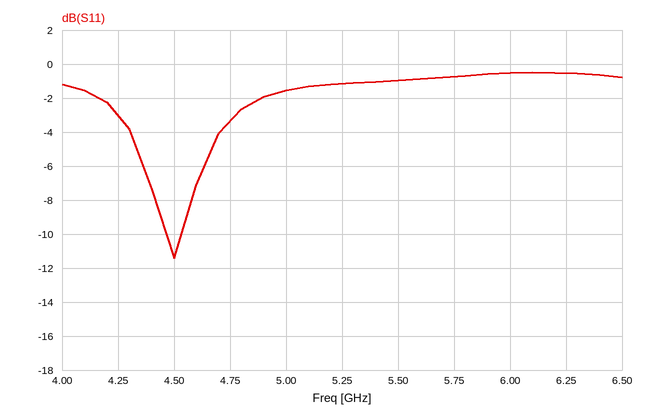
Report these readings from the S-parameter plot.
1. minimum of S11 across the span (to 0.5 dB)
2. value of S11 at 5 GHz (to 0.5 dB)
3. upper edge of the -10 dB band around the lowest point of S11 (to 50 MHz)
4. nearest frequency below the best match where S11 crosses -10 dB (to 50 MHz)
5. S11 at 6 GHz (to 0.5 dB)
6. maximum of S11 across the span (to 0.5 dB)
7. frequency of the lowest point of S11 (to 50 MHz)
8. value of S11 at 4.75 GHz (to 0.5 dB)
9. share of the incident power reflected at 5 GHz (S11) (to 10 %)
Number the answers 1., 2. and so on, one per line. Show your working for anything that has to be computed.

1. -11.5 dB
2. -1.5 dB
3. 4.55 GHz
4. 4.45 GHz
5. -0.5 dB
6. -0.5 dB
7. 4.50 GHz
8. -3.5 dB
9. 10^(-1.5/10) ≈ 70.8 %, so 70 % to the nearest 10 %
